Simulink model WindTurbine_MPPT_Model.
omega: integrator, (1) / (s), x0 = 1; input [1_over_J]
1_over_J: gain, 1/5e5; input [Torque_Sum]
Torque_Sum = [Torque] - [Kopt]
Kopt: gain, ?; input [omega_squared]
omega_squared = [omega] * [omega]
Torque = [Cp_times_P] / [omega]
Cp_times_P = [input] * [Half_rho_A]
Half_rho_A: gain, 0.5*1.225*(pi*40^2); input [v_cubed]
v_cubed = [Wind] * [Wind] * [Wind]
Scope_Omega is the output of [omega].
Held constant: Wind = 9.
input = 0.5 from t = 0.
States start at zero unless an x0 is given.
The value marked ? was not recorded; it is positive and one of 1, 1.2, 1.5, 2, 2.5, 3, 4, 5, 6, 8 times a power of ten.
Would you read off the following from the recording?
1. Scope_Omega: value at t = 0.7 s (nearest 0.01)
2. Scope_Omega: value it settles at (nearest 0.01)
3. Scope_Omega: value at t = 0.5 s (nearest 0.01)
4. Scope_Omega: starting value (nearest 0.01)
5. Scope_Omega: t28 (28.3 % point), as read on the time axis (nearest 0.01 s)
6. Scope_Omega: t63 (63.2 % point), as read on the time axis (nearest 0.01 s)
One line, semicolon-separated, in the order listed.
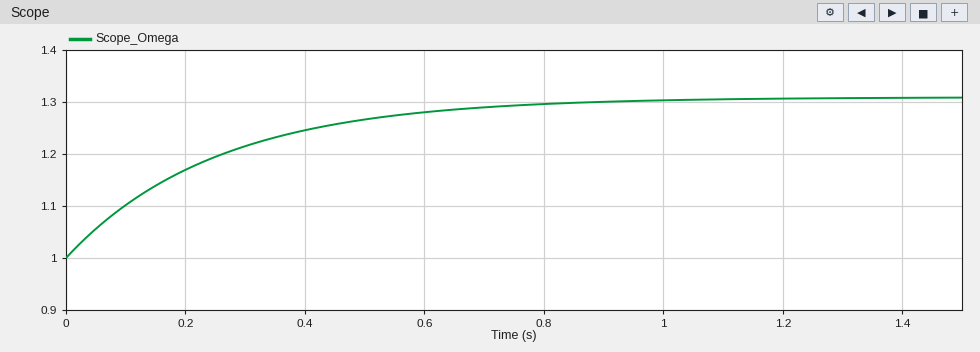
1.29; 1.31; 1.27; 1.00; 0.08 s; 0.25 s
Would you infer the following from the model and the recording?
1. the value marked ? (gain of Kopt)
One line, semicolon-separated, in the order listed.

500000
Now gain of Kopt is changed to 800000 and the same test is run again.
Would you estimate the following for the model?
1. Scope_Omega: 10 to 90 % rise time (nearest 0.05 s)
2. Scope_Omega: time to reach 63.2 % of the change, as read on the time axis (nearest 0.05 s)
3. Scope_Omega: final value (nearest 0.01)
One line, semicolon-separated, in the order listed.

0.40 s; 0.20 s; 1.12
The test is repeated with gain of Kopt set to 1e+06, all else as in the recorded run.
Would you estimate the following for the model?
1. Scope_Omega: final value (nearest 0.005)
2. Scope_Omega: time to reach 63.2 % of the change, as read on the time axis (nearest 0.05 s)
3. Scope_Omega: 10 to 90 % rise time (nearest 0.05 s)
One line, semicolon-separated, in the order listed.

1.040; 0.15 s; 0.35 s
